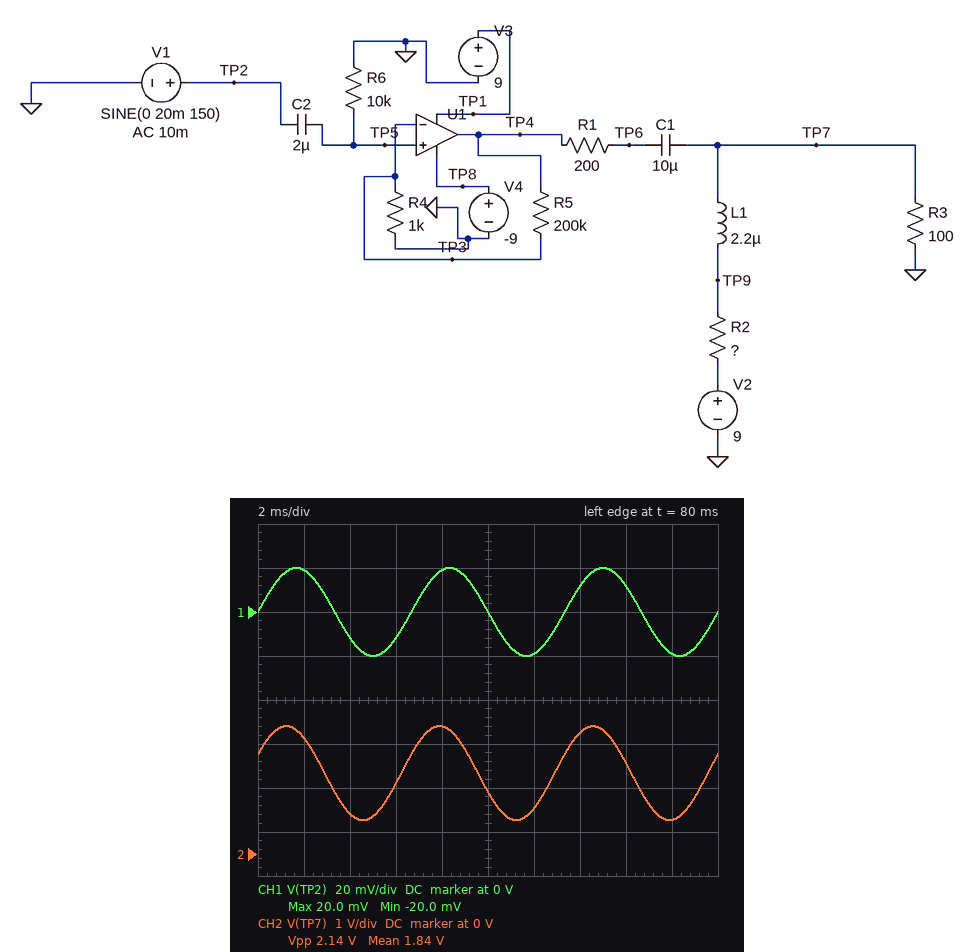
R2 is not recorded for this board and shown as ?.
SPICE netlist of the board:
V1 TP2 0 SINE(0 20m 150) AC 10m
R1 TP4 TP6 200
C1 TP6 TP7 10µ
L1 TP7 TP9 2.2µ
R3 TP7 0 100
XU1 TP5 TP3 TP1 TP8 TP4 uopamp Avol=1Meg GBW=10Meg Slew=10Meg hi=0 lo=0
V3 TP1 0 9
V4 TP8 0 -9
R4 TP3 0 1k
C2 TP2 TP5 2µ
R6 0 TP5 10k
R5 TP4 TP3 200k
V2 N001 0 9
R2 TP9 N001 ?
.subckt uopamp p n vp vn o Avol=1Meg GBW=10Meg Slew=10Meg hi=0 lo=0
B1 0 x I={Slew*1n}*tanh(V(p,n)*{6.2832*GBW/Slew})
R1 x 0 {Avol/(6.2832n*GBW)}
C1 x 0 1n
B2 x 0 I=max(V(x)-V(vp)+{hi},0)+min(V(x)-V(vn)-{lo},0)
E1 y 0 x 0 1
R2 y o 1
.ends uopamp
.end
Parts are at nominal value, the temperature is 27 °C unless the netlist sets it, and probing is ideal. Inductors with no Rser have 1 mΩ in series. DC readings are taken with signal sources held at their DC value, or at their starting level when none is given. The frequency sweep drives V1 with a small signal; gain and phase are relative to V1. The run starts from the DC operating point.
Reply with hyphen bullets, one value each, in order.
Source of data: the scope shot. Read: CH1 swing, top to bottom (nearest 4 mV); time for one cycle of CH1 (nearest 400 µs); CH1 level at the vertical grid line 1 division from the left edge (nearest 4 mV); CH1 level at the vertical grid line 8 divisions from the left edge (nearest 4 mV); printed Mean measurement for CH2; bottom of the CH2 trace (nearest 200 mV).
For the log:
- 40 mV
- 6.8 ms
- 20 mV
- 12 mV
- 1.84 V
- 800 mV
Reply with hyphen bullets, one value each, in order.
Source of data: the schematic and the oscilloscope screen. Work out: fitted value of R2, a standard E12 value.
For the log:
- 390 Ω
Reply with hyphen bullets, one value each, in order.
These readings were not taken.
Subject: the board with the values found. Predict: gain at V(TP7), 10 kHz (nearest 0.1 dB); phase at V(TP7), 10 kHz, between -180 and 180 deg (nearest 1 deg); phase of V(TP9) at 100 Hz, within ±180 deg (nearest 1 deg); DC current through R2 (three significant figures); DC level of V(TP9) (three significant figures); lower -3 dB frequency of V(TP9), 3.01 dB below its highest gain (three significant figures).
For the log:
- 35.0 dB
- -11 deg
- 34 deg
- 18.4 mA
- 1.84 V
- 57.9 Hz
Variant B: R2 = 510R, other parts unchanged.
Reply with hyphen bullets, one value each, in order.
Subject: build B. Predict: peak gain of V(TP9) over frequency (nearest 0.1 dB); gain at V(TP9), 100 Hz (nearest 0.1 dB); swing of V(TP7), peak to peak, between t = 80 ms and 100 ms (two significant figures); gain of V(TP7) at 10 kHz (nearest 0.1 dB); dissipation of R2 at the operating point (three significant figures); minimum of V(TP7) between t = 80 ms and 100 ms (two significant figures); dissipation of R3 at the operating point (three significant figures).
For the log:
- 35.4 dB
- 34.2 dB
- 2.2 V
- 35.3 dB
- 111 mW
- 370 mV
- 21.8 mW
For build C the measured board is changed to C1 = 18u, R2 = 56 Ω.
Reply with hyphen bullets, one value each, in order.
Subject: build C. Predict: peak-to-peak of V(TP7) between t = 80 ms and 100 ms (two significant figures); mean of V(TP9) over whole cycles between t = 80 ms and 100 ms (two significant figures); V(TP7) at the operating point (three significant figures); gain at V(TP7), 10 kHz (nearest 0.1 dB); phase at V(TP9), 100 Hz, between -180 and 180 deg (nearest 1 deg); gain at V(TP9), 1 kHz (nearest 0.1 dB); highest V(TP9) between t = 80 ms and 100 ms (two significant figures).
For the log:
- 1.2 V
- 5.8 V
- 5.77 V
- 29.5 dB
- 25 deg
- 29.7 dB
- 6.4 V
